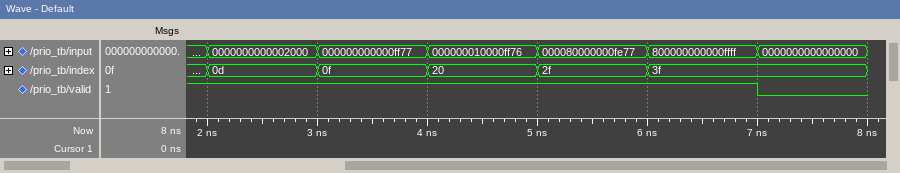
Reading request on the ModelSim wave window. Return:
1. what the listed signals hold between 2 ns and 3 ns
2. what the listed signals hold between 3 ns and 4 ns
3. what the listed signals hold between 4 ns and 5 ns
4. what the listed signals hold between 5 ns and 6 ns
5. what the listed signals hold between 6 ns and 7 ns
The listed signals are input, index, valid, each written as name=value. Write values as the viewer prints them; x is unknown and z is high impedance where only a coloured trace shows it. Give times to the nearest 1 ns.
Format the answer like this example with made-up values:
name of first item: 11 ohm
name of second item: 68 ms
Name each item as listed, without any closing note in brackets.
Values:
what the listed signals hold between 2 ns and 3 ns: input=0000000000002000, index=0d, valid=1
what the listed signals hold between 3 ns and 4 ns: input=000000000000ff77, index=0f, valid=1
what the listed signals hold between 4 ns and 5 ns: input=000000010000ff76, index=20, valid=1
what the listed signals hold between 5 ns and 6 ns: input=000080000000fe77, index=2f, valid=1
what the listed signals hold between 6 ns and 7 ns: input=800000000000ffff, index=3f, valid=1
